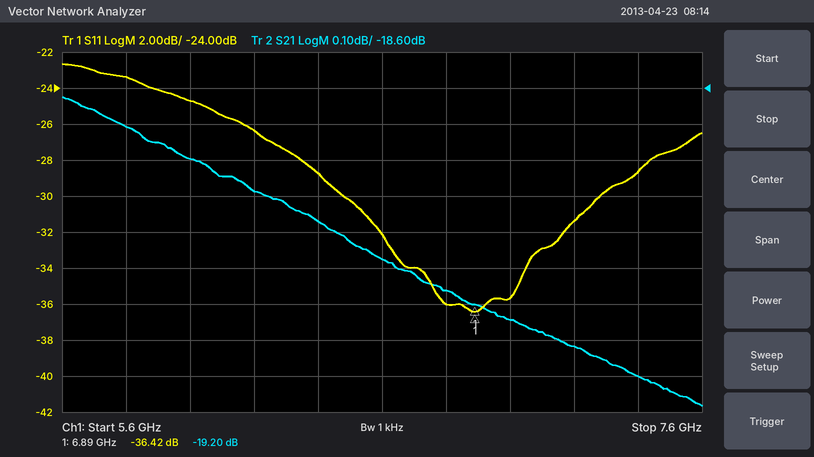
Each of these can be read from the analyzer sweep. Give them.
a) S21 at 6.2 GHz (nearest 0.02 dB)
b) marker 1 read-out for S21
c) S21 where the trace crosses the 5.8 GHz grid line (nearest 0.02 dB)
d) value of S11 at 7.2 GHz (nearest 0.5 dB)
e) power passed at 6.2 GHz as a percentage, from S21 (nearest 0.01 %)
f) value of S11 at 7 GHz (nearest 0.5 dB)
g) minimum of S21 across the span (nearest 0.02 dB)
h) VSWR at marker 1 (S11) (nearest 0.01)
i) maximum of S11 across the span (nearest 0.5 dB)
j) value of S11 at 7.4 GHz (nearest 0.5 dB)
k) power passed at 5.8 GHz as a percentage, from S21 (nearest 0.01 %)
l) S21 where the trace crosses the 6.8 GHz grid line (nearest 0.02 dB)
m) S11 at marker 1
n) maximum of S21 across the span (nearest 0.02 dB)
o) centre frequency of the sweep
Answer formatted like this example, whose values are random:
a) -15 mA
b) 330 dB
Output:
a) -18.88 dB
b) -19.20 dB
c) -18.70 dB
d) -31.5 dB
e) 1.29 %
f) -35.5 dB
g) -19.48 dB
h) 1.03
i) -22.5 dB
j) -28.5 dB
k) 1.35 %
l) -19.16 dB
m) -36.42 dB
n) -18.62 dB
o) 6.6 GHz
